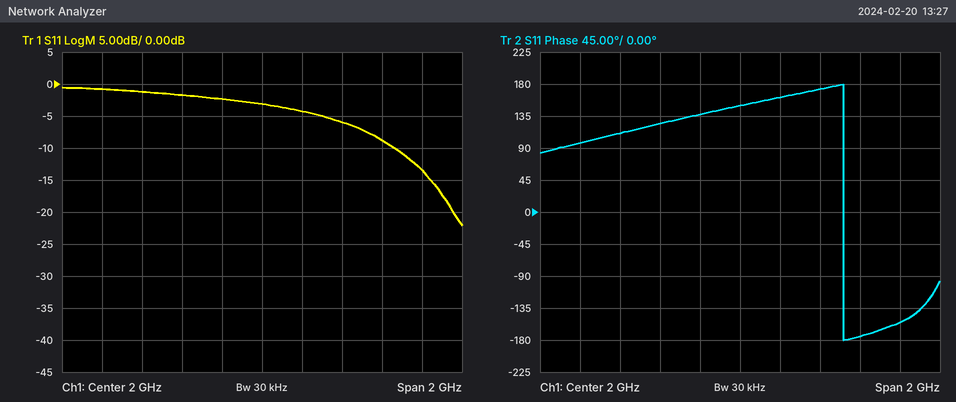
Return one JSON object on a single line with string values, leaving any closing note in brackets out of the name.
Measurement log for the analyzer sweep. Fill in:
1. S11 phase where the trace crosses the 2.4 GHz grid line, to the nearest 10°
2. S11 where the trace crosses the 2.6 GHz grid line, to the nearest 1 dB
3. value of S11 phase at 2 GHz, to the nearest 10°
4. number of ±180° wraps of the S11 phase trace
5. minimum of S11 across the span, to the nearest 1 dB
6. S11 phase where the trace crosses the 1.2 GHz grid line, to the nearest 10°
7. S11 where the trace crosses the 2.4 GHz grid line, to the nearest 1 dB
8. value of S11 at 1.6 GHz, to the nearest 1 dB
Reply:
{"S11 phase where the trace crosses the 2.4 GHz grid line, to the nearest 10°": "170°", "S11 where the trace crosses the 2.6 GHz grid line, to the nearest 1 dB": "-9 dB", "value of S11 phase at 2 GHz, to the nearest 10°": "150°", "number of ±180° wraps of the S11 phase trace": "1", "minimum of S11 across the span, to the nearest 1 dB": "-22 dB", "S11 phase where the trace crosses the 1.2 GHz grid line, to the nearest 10°": "100°", "S11 where the trace crosses the 2.4 GHz grid line, to the nearest 1 dB": "-6 dB", "value of S11 at 1.6 GHz, to the nearest 1 dB": "-2 dB"}
